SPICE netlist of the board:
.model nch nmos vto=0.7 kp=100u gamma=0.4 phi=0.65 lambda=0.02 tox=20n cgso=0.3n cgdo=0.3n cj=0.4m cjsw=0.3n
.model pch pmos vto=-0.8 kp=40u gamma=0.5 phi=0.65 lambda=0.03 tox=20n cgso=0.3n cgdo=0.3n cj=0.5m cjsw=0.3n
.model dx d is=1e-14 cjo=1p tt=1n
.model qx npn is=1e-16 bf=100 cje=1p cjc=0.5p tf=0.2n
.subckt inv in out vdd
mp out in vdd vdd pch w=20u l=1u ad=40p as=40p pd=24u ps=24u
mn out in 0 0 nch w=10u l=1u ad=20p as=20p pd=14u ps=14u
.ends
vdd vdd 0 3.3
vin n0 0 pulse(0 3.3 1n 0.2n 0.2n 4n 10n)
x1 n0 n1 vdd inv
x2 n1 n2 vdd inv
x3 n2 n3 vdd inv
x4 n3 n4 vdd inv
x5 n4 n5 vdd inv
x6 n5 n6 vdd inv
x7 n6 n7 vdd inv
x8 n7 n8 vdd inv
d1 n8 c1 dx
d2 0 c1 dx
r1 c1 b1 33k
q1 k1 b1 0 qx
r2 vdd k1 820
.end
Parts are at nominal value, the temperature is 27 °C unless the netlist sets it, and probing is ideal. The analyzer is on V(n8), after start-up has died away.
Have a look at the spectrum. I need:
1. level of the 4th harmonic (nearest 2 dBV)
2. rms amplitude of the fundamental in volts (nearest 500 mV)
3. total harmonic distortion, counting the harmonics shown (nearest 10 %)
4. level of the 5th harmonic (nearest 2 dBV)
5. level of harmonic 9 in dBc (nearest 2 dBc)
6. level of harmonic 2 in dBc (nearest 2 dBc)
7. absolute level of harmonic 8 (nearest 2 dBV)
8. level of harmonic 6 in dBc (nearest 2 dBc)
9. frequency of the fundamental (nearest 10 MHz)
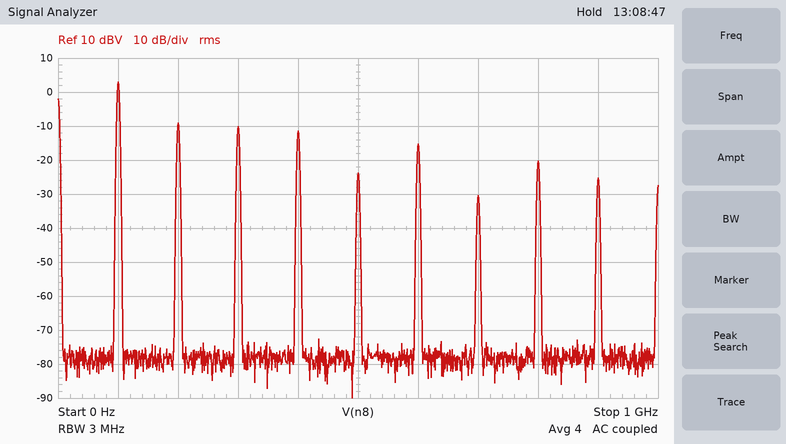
-12 dBV
1.5 V
40 %
-24 dBV
-28 dBc
-12 dBc
-20 dBV
-18 dBc
100 MHz
